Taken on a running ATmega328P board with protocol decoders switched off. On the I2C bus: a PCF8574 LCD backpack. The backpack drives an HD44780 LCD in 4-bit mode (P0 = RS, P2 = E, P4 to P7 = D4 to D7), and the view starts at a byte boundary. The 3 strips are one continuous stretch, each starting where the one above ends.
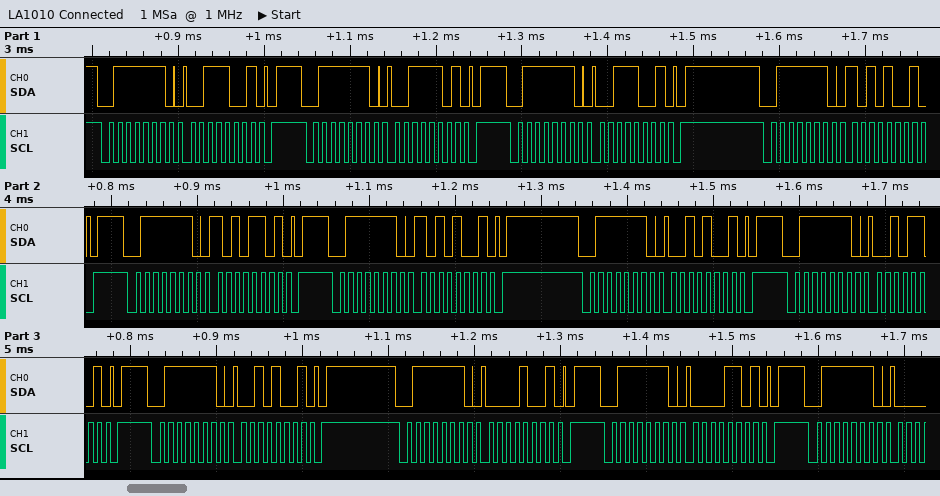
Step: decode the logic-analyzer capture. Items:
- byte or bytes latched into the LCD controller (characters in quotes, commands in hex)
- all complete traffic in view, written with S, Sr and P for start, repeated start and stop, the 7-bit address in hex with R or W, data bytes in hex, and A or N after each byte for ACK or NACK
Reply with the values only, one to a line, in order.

':'
S 3FW A 39 A P S 3FW A 3D A P S 3FW A 39 A P S 3FW A A9 A P S 3FW A AD A P S 3FW A A9 A P S 3FW A 29 A P S 3FW A 2D A P S 3FW A 29 A P S 3FW A 09 A P S 3FW A 0D A P S 3FW A
